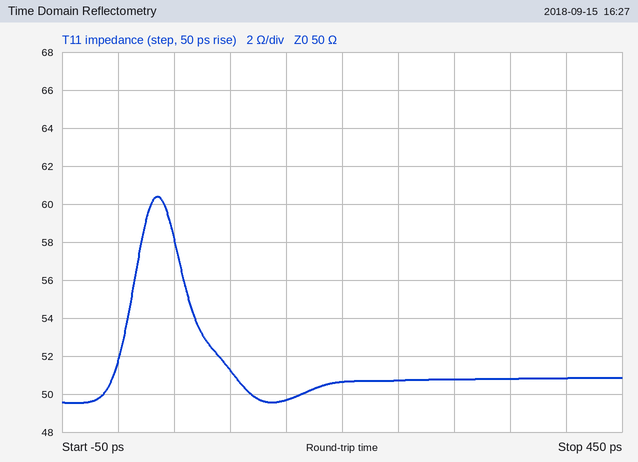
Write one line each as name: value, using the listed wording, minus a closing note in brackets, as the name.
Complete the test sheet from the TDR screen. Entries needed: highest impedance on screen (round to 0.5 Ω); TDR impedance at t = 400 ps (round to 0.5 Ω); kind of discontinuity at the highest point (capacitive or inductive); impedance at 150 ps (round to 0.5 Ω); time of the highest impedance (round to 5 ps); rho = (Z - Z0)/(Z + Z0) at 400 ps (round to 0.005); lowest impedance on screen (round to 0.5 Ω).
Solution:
highest impedance on screen: 60.5 Ω
TDR impedance at t = 400 ps: 51.0 Ω
kind of discontinuity at the highest point: inductive
impedance at 150 ps: 49.5 Ω
time of the highest impedance: 35 ps
rho = (Z - Z0)/(Z + Z0) at 400 ps: +0.010
lowest impedance on screen: 49.5 Ω
